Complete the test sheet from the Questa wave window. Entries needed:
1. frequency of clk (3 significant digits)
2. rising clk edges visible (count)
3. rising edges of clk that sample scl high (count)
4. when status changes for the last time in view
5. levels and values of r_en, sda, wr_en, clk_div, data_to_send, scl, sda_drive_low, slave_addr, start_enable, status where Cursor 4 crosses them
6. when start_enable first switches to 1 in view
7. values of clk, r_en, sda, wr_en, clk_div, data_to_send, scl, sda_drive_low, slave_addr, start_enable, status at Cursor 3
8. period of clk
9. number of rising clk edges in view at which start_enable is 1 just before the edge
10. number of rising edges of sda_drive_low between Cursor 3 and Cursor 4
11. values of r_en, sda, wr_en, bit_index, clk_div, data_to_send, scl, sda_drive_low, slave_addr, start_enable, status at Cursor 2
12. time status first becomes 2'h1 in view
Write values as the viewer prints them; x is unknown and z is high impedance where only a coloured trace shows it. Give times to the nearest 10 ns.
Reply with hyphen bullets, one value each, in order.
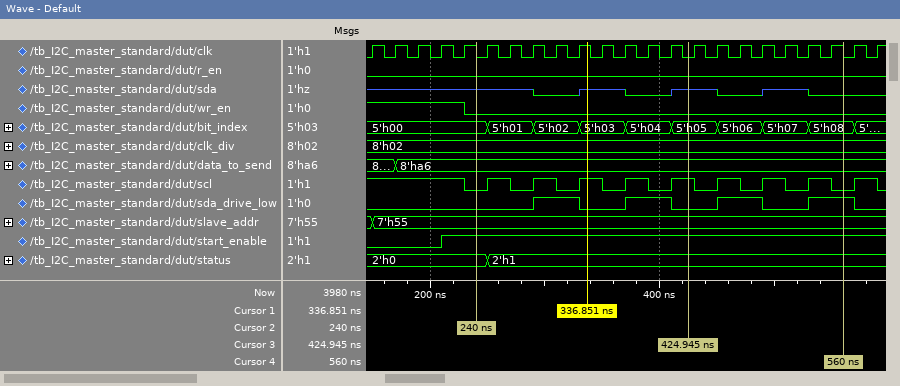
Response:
- 50.0 MHz
- 23
- 14
- 250 ns
- r_en=0, sda=0, wr_en=0, clk_div=8'h02, data_to_send=8'ha6, scl=0, sda_drive_low=1, slave_addr=7'h55, start_enable=1, status=2'h1
- 210 ns
- clk=0, r_en=0, sda=z, wr_en=0, clk_div=8'h02, data_to_send=8'ha6, scl=1, sda_drive_low=0, slave_addr=7'h55, start_enable=1, status=2'h1
- 20 ns
- 19
- 2
- r_en=0, sda=z, wr_en=0, bit_index=5'h00, clk_div=8'h02, data_to_send=8'ha6, scl=0, sda_drive_low=0, slave_addr=7'h55, start_enable=1, status=2'h0
- 250 ns
